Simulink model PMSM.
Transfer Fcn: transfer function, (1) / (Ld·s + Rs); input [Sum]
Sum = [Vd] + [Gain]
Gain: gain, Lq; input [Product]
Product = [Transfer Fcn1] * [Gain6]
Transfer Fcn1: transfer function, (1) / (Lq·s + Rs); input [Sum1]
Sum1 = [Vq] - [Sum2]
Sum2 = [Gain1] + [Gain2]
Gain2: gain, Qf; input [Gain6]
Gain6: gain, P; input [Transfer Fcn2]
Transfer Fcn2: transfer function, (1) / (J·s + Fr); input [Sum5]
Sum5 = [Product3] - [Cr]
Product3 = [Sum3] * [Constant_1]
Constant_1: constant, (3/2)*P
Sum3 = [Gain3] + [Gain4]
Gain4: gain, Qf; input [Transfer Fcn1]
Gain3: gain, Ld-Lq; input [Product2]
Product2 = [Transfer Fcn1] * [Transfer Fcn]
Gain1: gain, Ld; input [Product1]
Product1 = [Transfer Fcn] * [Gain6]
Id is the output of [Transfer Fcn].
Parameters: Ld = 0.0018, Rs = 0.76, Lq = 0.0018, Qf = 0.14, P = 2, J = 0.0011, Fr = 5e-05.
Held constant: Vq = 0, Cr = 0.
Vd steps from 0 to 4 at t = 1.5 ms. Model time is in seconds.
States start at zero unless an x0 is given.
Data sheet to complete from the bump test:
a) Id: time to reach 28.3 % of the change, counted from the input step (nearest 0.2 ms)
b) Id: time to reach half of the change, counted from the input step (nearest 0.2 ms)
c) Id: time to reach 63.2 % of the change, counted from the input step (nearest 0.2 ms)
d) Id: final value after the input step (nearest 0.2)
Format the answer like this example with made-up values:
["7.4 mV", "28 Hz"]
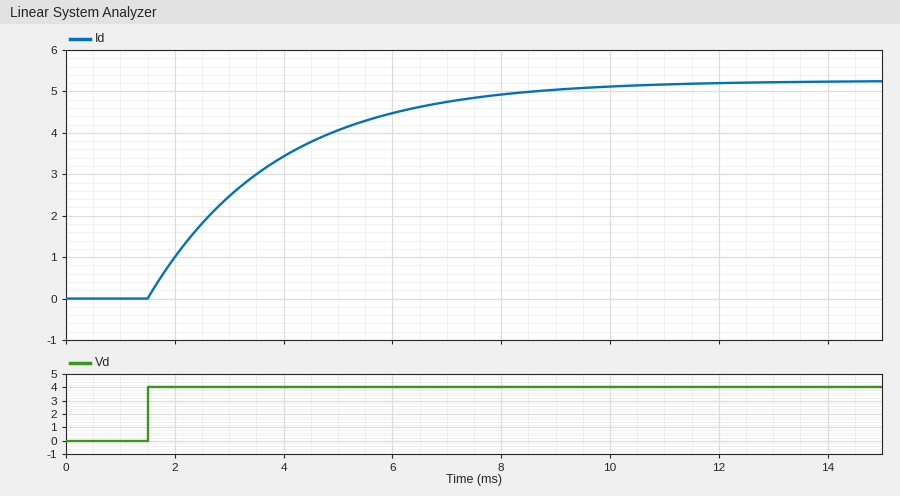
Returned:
["0.8 ms", "1.6 ms", "2.4 ms", "5.2"]
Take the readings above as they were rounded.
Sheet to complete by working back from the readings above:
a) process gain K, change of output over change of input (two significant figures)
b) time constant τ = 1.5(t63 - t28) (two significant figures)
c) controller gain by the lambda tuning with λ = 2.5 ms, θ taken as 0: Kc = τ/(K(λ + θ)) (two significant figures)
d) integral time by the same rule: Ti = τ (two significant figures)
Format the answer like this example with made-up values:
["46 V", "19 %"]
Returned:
["1.3", "2.4 ms", "0.74", "2.4 ms"]
